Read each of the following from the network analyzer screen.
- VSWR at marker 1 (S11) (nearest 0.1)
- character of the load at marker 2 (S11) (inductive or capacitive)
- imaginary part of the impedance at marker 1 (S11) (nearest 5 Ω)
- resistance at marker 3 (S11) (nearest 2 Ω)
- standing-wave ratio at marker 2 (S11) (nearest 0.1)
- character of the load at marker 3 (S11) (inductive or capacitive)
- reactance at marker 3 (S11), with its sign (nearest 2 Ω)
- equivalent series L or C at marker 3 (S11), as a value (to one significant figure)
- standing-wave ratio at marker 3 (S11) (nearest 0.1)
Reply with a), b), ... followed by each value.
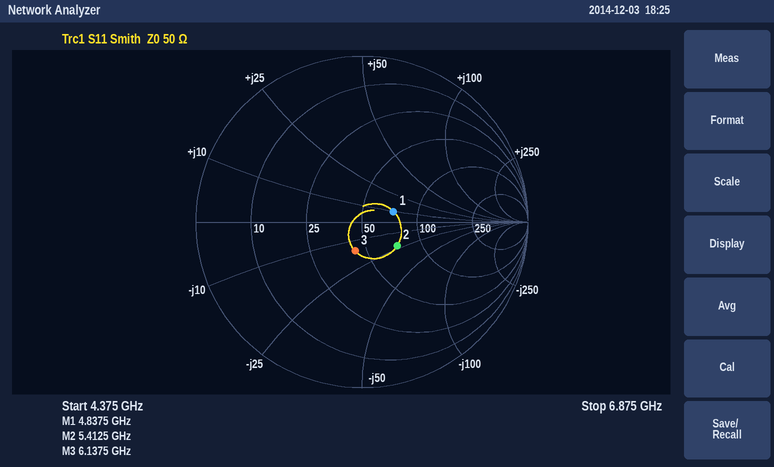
a) 1.5
b) capacitive
c) +10 Ω
d) 44 Ω
e) 1.7
f) capacitive
g) -16 Ω
h) 2 pF
i) 1.4
